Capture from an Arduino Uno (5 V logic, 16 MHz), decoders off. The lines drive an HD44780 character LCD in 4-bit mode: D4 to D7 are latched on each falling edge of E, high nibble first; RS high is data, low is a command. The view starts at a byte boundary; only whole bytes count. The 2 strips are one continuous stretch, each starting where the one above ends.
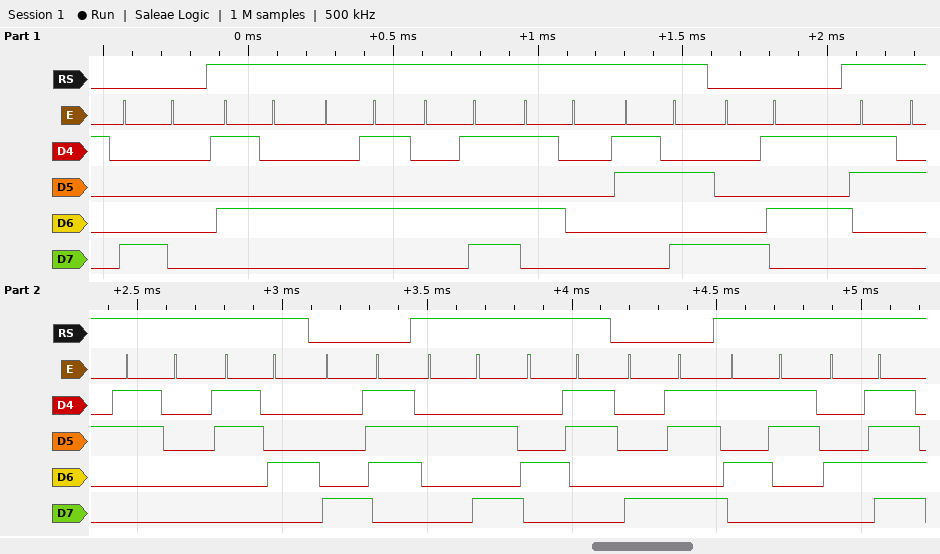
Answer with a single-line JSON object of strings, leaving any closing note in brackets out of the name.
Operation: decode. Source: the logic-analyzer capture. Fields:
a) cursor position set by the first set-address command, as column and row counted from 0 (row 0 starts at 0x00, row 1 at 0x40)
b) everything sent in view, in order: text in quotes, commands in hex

{"cursor position set by the first set-address command, as column and row counted from 0": "column 0, row 0", "everything sent in view, in order: text in quotes, commands in hex": "0x80 \"TEMP:\" 0x85 \"204\" 0x87 \"*C\" 0x8B \"SO\""}
